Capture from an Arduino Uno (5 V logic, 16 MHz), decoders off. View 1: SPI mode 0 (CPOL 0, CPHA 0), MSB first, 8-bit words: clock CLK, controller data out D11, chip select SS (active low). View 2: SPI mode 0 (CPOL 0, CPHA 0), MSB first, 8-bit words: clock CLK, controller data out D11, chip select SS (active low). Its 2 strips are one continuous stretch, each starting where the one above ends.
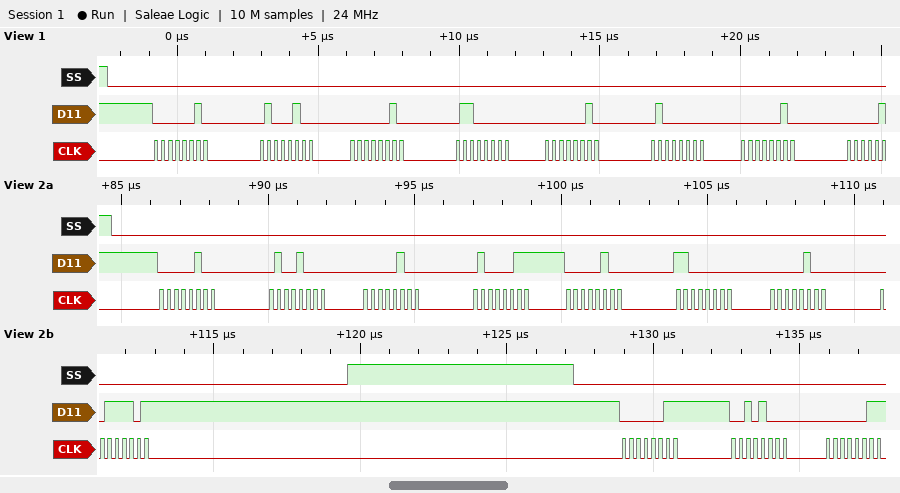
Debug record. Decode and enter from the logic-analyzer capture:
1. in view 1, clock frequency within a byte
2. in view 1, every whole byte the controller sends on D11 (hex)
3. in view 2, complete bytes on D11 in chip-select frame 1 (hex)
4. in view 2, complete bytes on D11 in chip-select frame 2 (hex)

4 MHz
02 44 02 60 02 40 02
04 48 04 43 04 C0 04 3D
03 28 03
